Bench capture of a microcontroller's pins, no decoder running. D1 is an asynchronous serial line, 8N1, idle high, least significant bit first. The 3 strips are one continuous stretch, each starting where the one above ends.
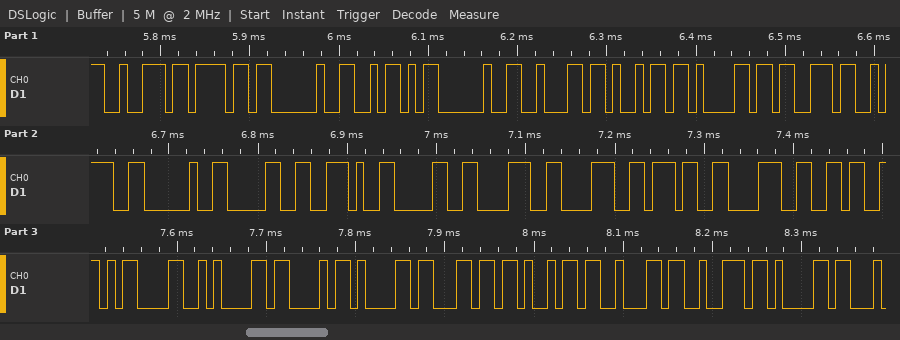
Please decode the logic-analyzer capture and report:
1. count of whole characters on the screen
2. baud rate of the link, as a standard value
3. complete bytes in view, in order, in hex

28
115200 baud
72 6F 20 5A 20 62 69 61 73 3A 20 30 2E 30 38 38 37 38 36 0D 0A 43 61 6C 69 62 72 61
